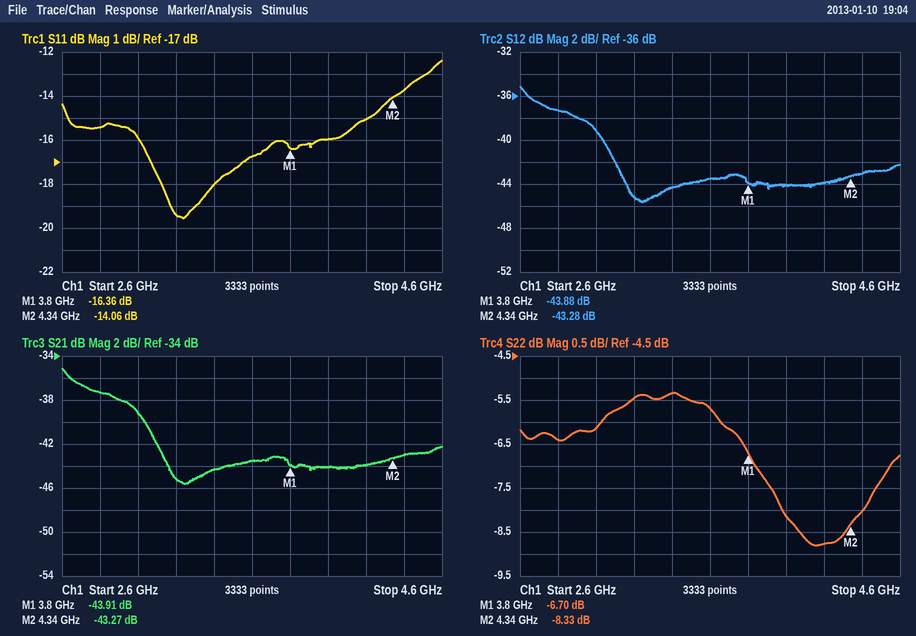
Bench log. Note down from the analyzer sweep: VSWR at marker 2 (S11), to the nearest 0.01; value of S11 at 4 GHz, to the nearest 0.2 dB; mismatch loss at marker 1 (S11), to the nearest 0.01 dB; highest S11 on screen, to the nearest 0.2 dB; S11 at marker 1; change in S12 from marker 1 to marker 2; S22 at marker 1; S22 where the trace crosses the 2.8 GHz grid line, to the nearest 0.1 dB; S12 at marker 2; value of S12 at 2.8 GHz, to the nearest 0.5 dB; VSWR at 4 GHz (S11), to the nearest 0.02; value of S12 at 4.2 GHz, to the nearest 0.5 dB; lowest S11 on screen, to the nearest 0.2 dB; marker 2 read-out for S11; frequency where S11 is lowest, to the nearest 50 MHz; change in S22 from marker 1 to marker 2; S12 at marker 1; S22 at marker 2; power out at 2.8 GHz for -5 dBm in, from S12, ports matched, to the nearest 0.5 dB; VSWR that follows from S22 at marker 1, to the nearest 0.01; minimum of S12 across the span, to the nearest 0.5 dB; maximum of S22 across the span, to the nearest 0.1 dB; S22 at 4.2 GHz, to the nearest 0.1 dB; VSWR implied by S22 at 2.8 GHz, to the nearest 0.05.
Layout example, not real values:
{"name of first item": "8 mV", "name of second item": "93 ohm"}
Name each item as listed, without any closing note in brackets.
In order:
{"VSWR at marker 2 (S11), to the nearest 0.01": "1.49", "value of S11 at 4 GHz, to the nearest 0.2 dB": "-16.0 dB", "mismatch loss at marker 1 (S11), to the nearest 0.01 dB": "0.10 dB", "highest S11 on screen, to the nearest 0.2 dB": "-12.4 dB", "S11 at marker 1": "-16.36 dB", "change in S12 from marker 1 to marker 2": "0.60 dB", "S22 at marker 1": "-6.70 dB", "S22 where the trace crosses the 2.8 GHz grid line, to the nearest 0.1 dB": "-6.4 dB", "S12 at marker 2": "-43.28 dB", "value of S12 at 2.8 GHz, to the nearest 0.5 dB": "-37.5 dB", "VSWR at 4 GHz (S11), to the nearest 0.02": "1.38", "value of S12 at 4.2 GHz, to the nearest 0.5 dB": "-44.0 dB", "lowest S11 on screen, to the nearest 0.2 dB": "-19.6 dB", "marker 2 read-out for S11": "-14.06 dB", "frequency where S11 is lowest, to the nearest 50 MHz": "3.25 GHz", "change in S22 from marker 1 to marker 2": "-1.63 dB", "S12 at marker 1": "-43.88 dB", "S22 at marker 2": "-8.33 dB", "power out at 2.8 GHz for -5 dBm in, from S12, ports matched, to the nearest 0.5 dB": "-42.5 dBm", "VSWR that follows from S22 at marker 1, to the nearest 0.01": "2.72", "minimum of S12 across the span, to the nearest 0.5 dB": "-45.5 dB", "maximum of S22 across the span, to the nearest 0.1 dB": "-5.3 dB", "S22 at 4.2 GHz, to the nearest 0.1 dB": "-8.8 dB", "VSWR implied by S22 at 2.8 GHz, to the nearest 0.05": "2.85"}
